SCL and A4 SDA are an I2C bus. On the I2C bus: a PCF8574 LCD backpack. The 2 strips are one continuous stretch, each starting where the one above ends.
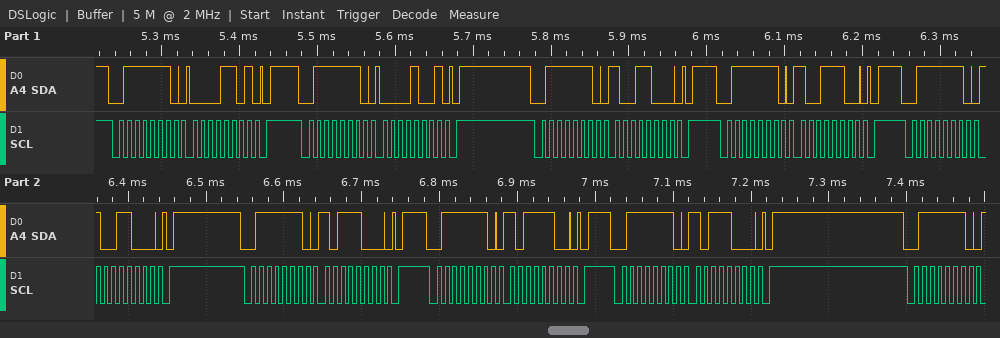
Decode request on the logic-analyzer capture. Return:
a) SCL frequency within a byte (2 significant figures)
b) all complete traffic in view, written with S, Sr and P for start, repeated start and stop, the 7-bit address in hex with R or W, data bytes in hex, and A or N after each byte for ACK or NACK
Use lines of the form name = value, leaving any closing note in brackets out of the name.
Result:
SCL frequency within a byte = 100 kHz
all complete traffic in view, written with S, Sr and P for start, repeated start and stop, the 7-bit address in hex with R or W, data bytes in hex, and A or N after each byte for ACK or NACK = S 3FW A 0D A P S 3FW A 09 A P S 3FW A 98 A P S 3FW A 9C A P S 3FW A 98 A P S 3FW A B8 A P S 3FW A BC A P S 3FW A B8 A P S 3FW A
